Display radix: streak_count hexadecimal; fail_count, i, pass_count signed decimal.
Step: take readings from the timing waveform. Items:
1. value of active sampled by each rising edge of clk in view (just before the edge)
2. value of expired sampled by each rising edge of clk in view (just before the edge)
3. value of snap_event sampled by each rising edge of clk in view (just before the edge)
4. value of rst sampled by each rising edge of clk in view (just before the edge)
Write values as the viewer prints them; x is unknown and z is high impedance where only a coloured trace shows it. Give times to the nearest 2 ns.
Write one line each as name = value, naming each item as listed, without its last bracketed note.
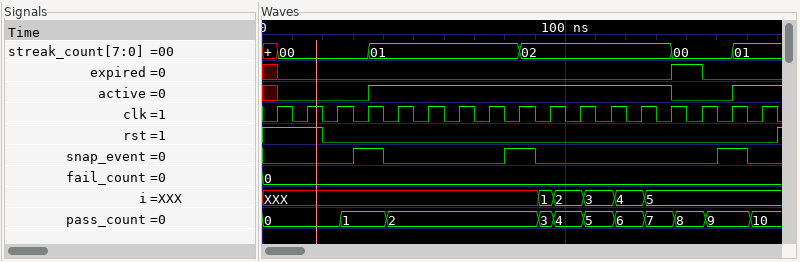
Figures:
value of active sampled by each rising edge of clk in view = x 0 0 0 1 1 1 1 1 1 1 1 1 1 0 0 1
value of expired sampled by each rising edge of clk in view = x 0 0 0 0 0 0 0 0 0 0 0 0 0 1 0 0
value of snap_event sampled by each rising edge of clk in view = 0 0 0 1 0 0 0 0 1 0 0 0 0 0 0 1 0
value of rst sampled by each rising edge of clk in view = 1 1 0 0 0 0 0 0 0 0 0 0 0 0 0 0 0
